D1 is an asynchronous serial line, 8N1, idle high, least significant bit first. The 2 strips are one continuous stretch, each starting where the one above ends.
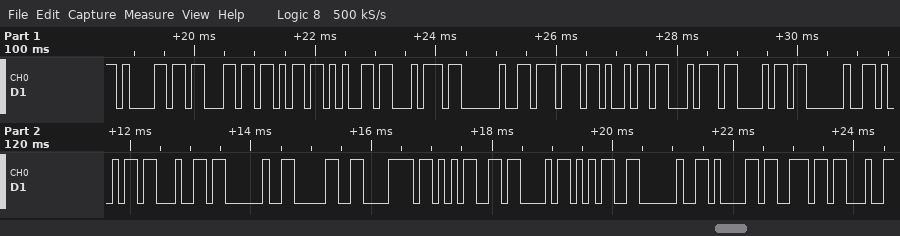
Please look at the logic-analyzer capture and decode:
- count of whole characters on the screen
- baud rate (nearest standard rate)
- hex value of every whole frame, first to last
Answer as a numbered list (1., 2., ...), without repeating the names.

1. 22
2. 9600 baud
3. 0x61 0x63 0x6B 0x65 0x74 0x20 0x77 0x69 0x74 0x68 0x20 0x69 0x64 0x20 0x30 0x78 0x35 0x43 0x35 0x20 0x61 0x6E
